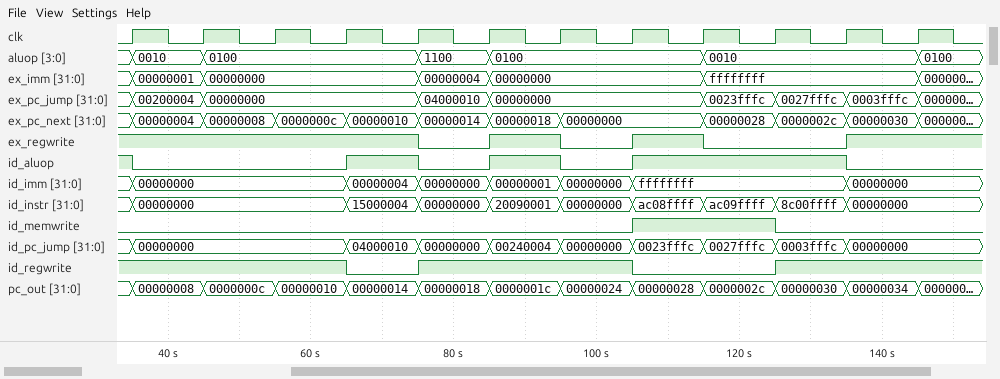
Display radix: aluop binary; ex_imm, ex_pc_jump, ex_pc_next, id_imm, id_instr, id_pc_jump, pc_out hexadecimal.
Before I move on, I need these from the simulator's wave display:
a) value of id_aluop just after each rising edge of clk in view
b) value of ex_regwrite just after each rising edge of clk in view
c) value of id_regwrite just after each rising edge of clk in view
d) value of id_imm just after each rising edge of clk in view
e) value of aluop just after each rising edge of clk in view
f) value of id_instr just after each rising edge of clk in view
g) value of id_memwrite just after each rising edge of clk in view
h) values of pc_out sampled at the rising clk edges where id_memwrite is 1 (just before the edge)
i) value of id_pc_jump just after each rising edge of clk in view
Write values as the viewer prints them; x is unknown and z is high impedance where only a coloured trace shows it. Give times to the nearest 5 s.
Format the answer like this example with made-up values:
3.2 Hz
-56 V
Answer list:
0 0 0 1 0 1 0 1 1 1 0 0
1 1 1 1 0 1 0 1 0 0 1 1
1 1 1 0 1 1 1 0 0 1 1 1
00000000, 00000000, 00000000, 00000004, 00000000, 00000001, 00000000, ffffffff, ffffffff, ffffffff, 00000000, 00000000
0010, 0100, 0100, 0100, 1100, 0100, 0100, 0100, 0010, 0010, 0010, 0100
00000000, 00000000, 00000000, 15000004, 00000000, 20090001, 00000000, ac08ffff, ac09ffff, 8c00ffff, 00000000, 00000000
0 0 0 0 0 0 0 1 1 0 0 0
00000028, 0000002c
00000000, 00000000, 00000000, 04000010, 00000000, 00240004, 00000000, 0023fffc, 0027fffc, 0003fffc, 00000000, 00000000
